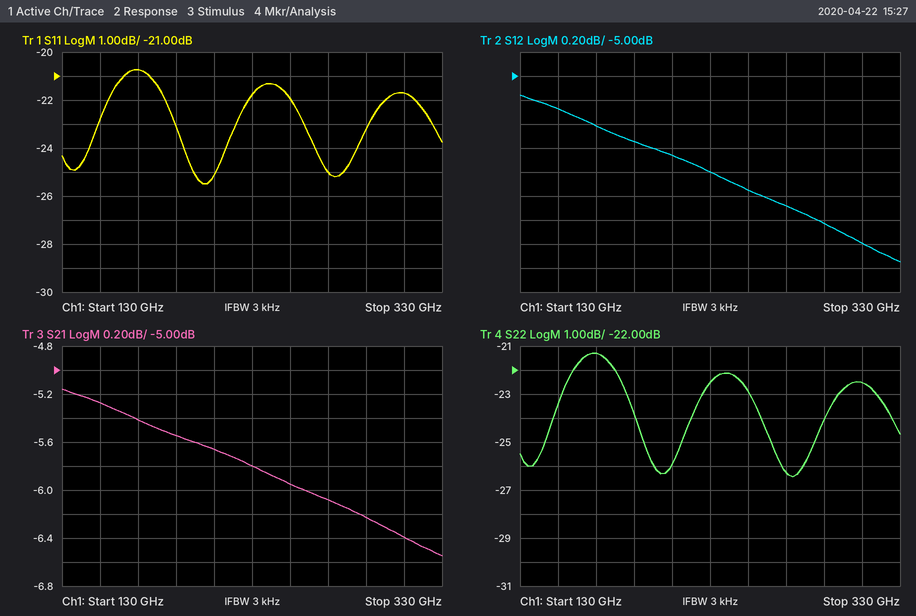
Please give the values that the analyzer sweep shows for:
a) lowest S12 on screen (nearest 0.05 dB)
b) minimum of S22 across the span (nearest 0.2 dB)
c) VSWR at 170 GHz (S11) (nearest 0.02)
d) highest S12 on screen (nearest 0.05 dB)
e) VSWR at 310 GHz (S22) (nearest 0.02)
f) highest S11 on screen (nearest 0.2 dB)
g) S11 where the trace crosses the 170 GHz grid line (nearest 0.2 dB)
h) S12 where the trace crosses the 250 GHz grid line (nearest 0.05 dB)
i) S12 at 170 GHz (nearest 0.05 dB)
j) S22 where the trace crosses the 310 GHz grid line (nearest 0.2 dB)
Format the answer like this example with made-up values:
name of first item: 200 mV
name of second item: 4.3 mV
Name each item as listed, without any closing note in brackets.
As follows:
lowest S12 on screen: -6.55 dB
minimum of S22 across the span: -26.4 dB
VSWR at 170 GHz (S11): 1.20
highest S12 on screen: -5.15 dB
VSWR at 310 GHz (S22): 1.16
highest S11 on screen: -20.8 dB
S11 where the trace crosses the 170 GHz grid line: -20.8 dB
S12 where the trace crosses the 250 GHz grid line: -5.95 dB
S12 at 170 GHz: -5.40 dB
S22 where the trace crosses the 310 GHz grid line: -22.6 dB
